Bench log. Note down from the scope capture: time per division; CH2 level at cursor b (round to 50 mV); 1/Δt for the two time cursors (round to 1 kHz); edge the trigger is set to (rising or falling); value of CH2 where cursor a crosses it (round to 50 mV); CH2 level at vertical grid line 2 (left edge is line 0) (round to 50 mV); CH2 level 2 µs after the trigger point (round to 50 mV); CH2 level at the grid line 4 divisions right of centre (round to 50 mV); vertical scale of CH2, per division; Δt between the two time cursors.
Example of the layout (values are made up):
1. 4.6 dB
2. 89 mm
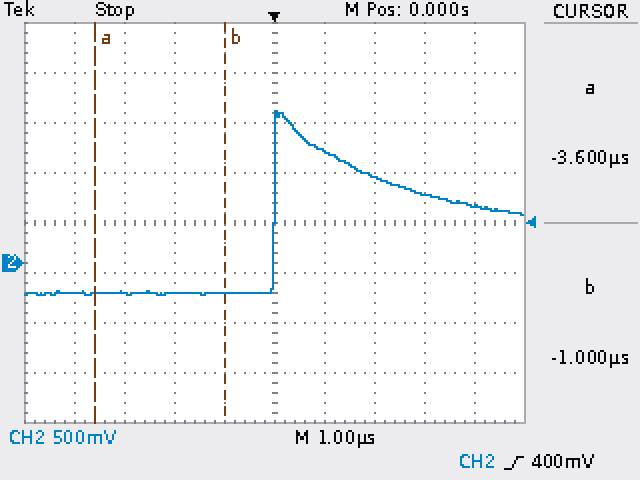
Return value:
1. 1 µs
2. -300 mV
3. 385 kHz
4. rising
5. -300 mV
6. -300 mV
7. 850 mV
8. 550 mV
9. 500 mV
10. 2.6 µs
